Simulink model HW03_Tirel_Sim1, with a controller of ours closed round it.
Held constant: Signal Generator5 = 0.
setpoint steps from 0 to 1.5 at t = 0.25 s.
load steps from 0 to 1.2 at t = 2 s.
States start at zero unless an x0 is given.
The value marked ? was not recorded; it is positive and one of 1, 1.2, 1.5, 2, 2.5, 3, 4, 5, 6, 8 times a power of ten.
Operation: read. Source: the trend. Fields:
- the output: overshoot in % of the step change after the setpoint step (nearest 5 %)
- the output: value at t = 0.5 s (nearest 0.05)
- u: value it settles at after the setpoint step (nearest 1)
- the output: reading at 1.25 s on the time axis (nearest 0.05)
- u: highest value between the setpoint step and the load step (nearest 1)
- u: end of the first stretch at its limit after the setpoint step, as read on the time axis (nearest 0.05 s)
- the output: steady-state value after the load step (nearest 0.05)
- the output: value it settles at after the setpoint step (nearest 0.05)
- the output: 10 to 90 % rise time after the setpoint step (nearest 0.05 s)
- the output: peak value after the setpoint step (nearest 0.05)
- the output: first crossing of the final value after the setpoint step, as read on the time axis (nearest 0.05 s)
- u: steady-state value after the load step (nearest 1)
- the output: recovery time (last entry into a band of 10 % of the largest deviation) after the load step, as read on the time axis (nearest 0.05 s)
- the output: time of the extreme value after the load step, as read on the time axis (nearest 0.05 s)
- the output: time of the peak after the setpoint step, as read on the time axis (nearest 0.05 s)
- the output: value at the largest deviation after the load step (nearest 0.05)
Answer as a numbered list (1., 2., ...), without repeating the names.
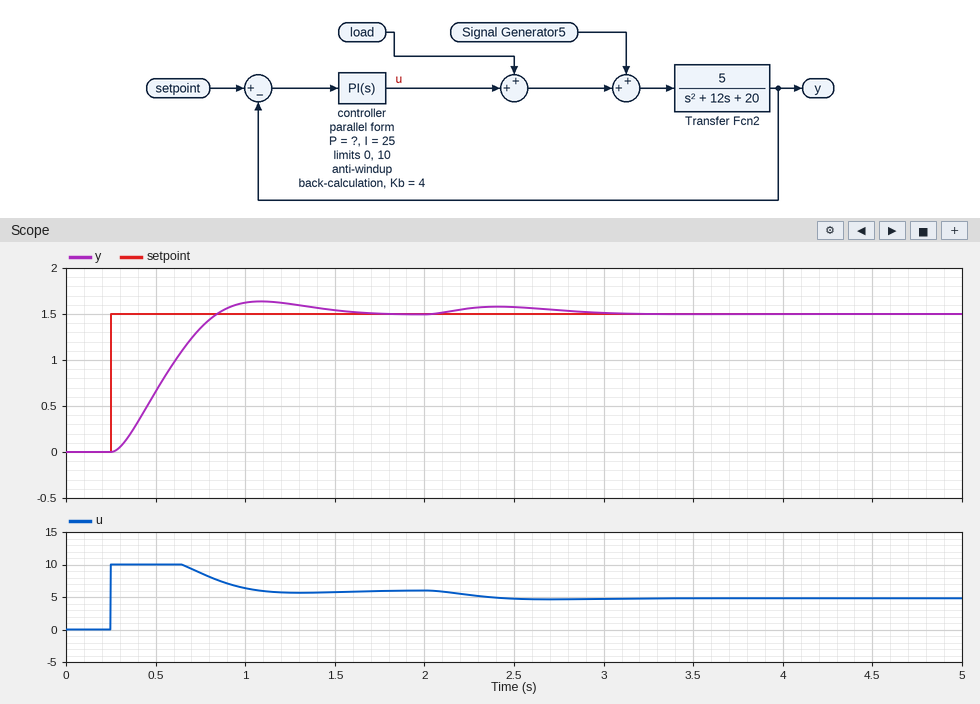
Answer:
1. 10 %
2. 0.65
3. 6
4. 1.60
5. 10
6. 0.65 s
7. 1.50
8. 1.50
9. 0.40 s
10. 1.65
11. 0.85 s
12. 5
13. 3.05 s
14. 2.40 s
15. 1.10 s
16. 1.60
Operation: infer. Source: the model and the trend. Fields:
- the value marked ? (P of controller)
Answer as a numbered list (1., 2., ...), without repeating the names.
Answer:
1. 8
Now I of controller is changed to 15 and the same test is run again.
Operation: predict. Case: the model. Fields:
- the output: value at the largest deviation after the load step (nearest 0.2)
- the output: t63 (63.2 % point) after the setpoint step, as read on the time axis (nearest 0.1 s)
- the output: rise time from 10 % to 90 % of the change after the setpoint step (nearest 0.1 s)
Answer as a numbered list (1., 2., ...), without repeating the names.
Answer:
1. 1.6
2. 0.6 s
3. 0.5 s
